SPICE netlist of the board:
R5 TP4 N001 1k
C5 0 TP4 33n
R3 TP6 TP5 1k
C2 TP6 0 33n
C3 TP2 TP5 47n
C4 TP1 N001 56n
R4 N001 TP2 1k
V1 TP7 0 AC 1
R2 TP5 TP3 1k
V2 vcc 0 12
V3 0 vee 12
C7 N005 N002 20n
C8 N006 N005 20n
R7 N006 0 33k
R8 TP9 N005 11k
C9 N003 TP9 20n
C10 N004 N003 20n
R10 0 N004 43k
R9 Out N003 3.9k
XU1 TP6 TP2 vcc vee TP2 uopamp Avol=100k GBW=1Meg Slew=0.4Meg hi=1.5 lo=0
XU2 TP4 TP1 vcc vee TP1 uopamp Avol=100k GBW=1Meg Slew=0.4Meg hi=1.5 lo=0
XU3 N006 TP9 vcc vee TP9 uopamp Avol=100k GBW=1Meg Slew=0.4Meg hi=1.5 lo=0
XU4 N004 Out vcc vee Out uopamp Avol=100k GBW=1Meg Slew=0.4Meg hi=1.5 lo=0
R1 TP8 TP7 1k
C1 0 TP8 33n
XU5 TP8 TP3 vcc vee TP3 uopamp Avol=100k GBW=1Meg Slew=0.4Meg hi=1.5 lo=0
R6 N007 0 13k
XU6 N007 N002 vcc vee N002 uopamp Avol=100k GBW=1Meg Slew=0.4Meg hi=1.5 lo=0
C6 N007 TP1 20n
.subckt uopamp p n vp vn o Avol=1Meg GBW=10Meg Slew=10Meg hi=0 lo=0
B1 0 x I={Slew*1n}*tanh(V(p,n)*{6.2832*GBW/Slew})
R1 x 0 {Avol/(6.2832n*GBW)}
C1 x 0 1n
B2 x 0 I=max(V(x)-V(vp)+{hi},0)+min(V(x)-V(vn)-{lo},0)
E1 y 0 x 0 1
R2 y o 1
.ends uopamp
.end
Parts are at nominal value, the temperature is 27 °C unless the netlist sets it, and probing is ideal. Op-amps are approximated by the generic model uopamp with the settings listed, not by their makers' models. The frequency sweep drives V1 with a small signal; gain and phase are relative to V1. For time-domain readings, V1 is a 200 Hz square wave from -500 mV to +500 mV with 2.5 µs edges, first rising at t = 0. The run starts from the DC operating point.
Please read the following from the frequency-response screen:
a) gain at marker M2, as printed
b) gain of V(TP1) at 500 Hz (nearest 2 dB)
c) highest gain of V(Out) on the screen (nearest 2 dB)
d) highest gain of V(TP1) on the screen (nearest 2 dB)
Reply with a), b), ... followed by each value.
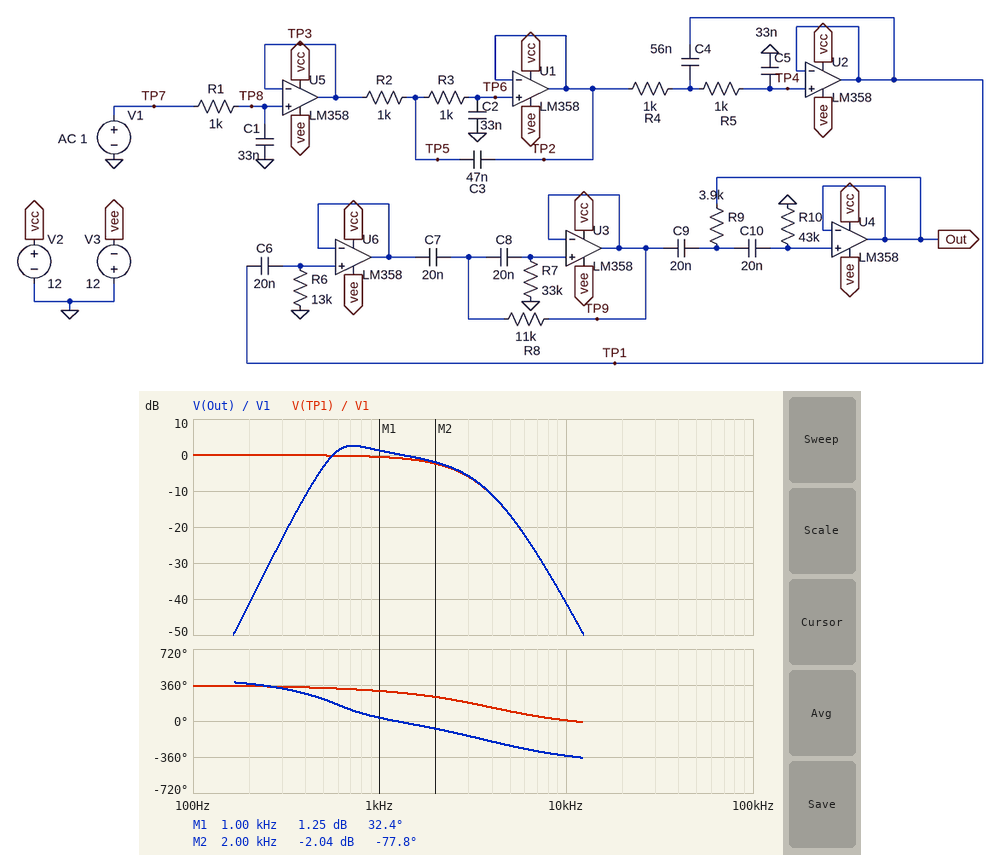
a) -2.04 dB
b) 0 dB
c) 2 dB
d) 0 dB
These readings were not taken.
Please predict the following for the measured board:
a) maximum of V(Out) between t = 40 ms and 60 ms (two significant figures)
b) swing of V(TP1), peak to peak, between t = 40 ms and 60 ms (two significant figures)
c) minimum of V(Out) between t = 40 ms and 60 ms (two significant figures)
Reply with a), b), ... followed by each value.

a) 470 mV
b) 1.0 V
c) -470 mV
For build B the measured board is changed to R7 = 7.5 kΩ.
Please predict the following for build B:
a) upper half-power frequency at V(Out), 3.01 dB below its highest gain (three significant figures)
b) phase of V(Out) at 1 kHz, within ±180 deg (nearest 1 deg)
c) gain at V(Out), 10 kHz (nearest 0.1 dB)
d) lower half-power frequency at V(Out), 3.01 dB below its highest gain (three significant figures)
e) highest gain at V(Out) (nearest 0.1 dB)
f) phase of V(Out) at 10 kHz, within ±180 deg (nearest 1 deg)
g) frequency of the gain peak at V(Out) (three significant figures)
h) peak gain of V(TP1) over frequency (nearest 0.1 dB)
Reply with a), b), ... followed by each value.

a) 3.08 kHz
b) 86 deg
c) -41.4 dB
d) 715 Hz
e) -4.5 dB
f) 22 deg
g) 1.72 kHz
h) 0 dB
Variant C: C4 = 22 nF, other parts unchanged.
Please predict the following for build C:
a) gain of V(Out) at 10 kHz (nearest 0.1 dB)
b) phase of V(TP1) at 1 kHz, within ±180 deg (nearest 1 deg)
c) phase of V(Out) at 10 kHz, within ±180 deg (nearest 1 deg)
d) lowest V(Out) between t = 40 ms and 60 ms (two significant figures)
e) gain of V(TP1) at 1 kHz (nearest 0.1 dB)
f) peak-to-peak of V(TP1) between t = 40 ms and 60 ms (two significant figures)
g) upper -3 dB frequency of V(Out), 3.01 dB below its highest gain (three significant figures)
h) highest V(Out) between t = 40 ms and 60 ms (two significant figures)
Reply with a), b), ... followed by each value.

a) -36.8 dB
b) -59 deg
c) 45 deg
d) -450 mV
e) -0.9 dB
f) 1.0 V
g) 1.34 kHz
h) 450 mV
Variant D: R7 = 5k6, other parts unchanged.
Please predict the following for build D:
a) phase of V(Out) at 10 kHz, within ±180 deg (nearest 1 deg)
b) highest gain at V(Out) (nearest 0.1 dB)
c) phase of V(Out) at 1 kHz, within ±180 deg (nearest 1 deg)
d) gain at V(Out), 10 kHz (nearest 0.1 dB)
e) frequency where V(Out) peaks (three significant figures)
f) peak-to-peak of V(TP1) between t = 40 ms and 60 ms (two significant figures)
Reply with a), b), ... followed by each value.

a) 26 deg
b) -6.2 dB
c) 93 deg
d) -41.5 dB
e) 1.93 kHz
f) 1.0 V
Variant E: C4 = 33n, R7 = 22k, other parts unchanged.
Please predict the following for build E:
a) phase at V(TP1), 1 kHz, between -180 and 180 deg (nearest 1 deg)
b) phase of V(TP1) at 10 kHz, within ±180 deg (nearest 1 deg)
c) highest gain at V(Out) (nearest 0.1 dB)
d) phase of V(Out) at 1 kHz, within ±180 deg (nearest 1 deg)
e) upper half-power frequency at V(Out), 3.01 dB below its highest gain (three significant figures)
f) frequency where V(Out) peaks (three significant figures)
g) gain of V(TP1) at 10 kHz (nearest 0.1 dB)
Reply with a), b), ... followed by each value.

a) -59 deg
b) 24 deg
c) 1.0 dB
d) 47 deg
e) 1.74 kHz
f) 764 Hz
g) -38.2 dB
